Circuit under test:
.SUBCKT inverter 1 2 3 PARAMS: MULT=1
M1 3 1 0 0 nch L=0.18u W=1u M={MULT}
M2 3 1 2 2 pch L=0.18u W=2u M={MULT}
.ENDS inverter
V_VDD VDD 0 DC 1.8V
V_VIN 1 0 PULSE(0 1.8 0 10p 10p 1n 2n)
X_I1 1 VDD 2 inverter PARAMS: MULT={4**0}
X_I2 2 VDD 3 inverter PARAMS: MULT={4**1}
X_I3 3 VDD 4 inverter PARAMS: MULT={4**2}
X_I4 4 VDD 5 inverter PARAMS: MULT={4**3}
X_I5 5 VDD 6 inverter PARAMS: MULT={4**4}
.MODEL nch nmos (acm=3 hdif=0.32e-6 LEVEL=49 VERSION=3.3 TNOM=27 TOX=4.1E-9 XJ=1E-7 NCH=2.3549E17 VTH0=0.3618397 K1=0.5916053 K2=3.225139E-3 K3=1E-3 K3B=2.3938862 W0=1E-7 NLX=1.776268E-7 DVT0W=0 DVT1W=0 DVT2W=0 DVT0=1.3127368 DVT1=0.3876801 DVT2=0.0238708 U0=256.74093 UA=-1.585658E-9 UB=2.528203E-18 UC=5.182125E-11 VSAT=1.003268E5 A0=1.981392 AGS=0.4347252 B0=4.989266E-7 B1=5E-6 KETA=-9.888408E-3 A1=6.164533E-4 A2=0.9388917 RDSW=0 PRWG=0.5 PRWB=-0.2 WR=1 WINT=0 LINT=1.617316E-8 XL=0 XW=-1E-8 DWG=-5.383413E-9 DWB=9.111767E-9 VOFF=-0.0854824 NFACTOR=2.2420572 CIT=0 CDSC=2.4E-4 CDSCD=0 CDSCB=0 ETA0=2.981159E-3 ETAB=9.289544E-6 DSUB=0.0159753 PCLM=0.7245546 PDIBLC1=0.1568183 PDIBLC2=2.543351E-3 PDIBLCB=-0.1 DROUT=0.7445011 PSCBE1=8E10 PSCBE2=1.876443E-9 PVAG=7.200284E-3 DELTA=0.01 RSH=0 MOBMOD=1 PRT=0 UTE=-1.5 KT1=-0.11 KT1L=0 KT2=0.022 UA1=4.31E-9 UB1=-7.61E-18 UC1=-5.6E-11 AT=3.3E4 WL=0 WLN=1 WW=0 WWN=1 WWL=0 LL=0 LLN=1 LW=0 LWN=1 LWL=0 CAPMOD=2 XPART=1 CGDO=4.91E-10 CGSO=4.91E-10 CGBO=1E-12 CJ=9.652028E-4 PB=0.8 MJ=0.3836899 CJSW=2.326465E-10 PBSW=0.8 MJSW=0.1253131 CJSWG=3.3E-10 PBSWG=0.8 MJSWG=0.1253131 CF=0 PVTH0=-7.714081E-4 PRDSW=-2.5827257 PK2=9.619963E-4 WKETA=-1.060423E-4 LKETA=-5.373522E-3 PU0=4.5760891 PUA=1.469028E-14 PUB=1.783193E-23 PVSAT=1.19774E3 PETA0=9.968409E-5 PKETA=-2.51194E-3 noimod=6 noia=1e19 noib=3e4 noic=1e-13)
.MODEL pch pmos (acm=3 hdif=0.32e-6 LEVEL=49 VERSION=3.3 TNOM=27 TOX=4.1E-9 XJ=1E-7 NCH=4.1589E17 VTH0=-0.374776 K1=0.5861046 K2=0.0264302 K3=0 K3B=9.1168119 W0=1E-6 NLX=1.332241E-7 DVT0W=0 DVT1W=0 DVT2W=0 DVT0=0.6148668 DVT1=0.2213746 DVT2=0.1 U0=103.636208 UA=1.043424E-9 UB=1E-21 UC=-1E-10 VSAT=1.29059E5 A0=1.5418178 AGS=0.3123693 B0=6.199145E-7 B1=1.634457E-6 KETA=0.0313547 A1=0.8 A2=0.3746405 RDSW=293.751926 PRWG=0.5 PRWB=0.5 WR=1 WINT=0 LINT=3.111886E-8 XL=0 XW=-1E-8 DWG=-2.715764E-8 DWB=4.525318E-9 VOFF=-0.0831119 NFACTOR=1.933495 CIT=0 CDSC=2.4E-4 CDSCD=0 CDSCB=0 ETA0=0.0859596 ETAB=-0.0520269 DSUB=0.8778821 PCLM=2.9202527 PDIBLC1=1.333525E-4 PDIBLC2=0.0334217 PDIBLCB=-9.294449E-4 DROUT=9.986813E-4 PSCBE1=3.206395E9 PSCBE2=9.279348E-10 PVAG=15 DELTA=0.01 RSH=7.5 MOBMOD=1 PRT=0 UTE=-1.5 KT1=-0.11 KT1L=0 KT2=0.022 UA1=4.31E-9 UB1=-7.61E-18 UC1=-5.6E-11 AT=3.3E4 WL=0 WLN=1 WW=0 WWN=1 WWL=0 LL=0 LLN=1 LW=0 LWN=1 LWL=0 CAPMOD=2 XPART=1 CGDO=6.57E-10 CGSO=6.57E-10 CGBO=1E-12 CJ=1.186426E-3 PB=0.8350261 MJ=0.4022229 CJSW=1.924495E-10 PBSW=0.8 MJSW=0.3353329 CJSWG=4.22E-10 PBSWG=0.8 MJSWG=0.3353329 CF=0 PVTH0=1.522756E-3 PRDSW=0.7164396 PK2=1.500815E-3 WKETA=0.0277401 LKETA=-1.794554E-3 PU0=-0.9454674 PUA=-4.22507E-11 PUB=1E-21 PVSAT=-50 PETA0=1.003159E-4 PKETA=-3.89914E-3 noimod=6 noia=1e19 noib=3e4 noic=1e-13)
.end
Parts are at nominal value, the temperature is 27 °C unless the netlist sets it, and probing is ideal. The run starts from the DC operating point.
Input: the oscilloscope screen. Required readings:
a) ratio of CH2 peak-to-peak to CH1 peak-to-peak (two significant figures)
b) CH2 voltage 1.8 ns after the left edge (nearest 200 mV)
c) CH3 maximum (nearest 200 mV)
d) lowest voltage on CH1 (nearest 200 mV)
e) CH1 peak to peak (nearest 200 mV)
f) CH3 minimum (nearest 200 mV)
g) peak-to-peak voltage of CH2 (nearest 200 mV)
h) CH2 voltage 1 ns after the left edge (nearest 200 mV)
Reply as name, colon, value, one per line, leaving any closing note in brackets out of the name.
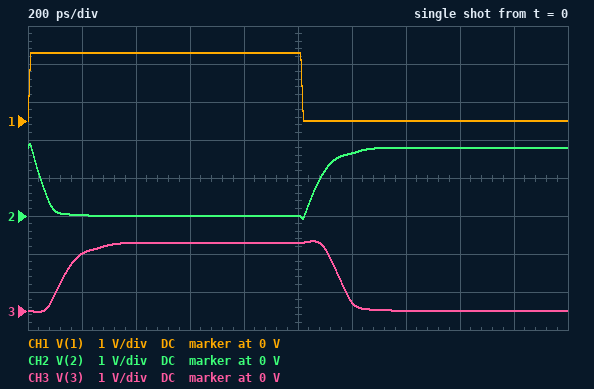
ratio of CH2 peak-to-peak to CH1 peak-to-peak: 1.1
CH2 voltage 1.8 ns after the left edge: 1.8 V
CH3 maximum: 1.8 V
lowest voltage on CH1: 0 V
CH1 peak to peak: 1.8 V
CH3 minimum: 0 V
peak-to-peak voltage of CH2: 2.0 V
CH2 voltage 1 ns after the left edge: 0 V
